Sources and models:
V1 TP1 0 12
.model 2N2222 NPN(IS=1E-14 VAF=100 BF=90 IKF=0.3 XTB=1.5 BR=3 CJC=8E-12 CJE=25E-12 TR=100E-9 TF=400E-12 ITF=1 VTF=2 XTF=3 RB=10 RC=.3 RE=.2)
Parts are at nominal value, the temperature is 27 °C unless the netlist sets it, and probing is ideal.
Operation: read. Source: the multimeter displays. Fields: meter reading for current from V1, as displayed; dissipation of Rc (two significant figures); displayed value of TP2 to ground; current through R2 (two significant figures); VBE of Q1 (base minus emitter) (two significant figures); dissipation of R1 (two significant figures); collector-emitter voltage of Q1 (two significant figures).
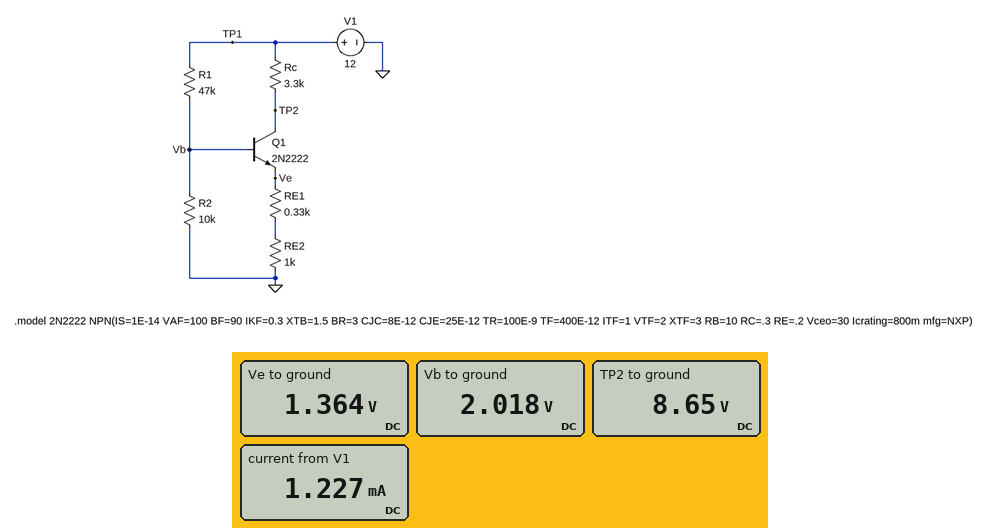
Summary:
1.227 mA
3.4 mW
8.65 V
200 µA
650 mV
2.1 mW
7.3 V
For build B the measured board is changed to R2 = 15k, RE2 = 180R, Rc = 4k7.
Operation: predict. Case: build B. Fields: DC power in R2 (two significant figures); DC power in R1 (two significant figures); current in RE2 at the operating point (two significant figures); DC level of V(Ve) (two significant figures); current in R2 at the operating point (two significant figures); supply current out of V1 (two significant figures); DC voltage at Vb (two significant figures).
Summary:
240 µW
2.2 mW
2.4 mA
1.2 V
130 µA
2.5 mA
1.9 V
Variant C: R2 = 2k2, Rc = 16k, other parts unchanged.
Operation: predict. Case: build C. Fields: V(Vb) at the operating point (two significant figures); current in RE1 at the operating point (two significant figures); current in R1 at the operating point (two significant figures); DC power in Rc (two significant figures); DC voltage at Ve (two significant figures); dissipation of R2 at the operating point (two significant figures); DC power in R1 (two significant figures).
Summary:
540 mV
7.7 µA
240 µA
930 nW
10 mV
130 µW
2.8 mW
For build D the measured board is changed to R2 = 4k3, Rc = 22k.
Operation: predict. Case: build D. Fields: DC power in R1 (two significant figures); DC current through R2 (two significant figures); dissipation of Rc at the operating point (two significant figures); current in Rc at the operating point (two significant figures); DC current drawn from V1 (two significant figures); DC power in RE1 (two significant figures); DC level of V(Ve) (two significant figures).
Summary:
2.6 mW
230 µA
1.7 mW
280 µA
510 µA
26 µW
370 mV
